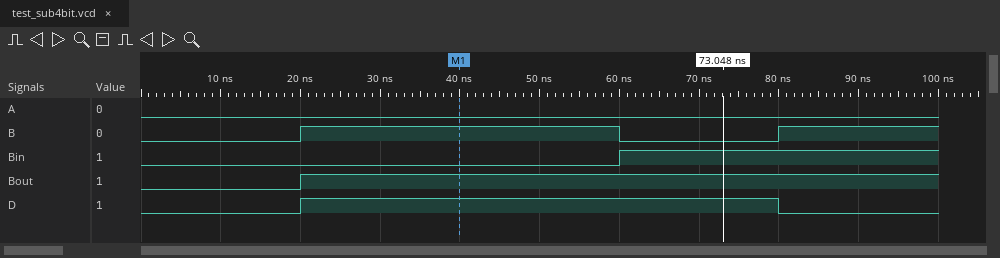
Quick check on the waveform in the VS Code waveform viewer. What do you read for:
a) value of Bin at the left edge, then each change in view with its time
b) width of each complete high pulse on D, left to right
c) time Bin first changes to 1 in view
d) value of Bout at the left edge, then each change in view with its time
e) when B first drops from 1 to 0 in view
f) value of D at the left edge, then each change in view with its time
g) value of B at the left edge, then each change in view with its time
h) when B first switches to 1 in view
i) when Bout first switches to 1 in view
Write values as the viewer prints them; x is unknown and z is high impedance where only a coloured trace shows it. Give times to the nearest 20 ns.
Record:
0, 1 at 60 ns
60 ns
60 ns
0, 1 at 20 ns
60 ns
0, 1 at 20 ns, 0 at 80 ns
0, 1 at 20 ns, 0 at 60 ns, 1 at 80 ns
20 ns
20 ns
